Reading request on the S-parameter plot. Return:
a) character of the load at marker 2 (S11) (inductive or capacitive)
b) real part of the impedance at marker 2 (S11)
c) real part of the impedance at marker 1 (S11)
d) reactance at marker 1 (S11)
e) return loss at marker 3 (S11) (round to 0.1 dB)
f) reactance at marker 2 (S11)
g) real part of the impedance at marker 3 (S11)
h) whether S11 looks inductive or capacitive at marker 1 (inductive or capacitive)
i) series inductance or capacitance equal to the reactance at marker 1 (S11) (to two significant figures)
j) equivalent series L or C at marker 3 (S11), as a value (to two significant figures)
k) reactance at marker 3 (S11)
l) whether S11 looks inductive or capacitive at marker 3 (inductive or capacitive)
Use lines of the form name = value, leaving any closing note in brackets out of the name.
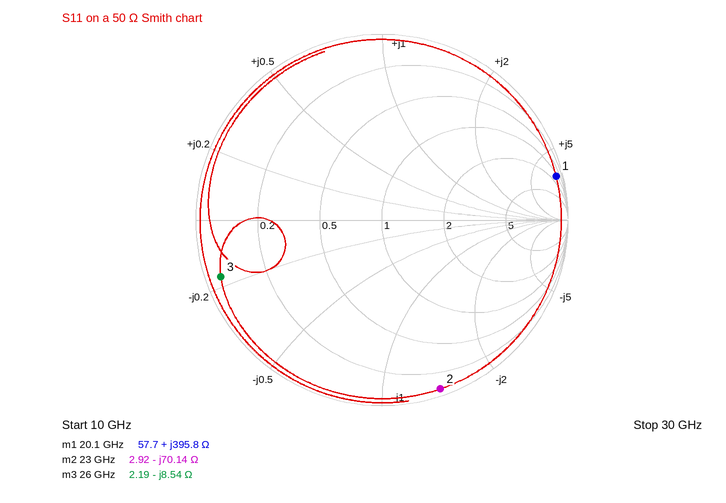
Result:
character of the load at marker 2 (S11) = capacitive
real part of the impedance at marker 2 = 2.92 Ω
real part of the impedance at marker 1 = 57.7 Ω
reactance at marker 1 = +395.8 Ω
return loss at marker 3 (S11) = 0.7 dB
reactance at marker 2 = -70.14 Ω
real part of the impedance at marker 3 = 2.19 Ω
whether S11 looks inductive or capacitive at marker 1 = inductive
series inductance or capacitance equal to the reactance at marker 1 (S11) = 3.1 nH
equivalent series L or C at marker 3 (S11), as a value = 720 fF
reactance at marker 3 = -8.54 Ω
whether S11 looks inductive or capacitive at marker 3 = capacitive
